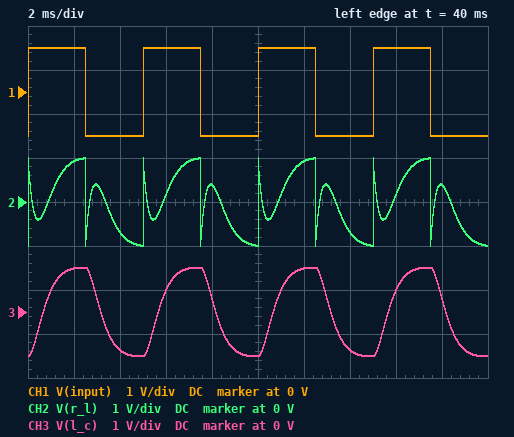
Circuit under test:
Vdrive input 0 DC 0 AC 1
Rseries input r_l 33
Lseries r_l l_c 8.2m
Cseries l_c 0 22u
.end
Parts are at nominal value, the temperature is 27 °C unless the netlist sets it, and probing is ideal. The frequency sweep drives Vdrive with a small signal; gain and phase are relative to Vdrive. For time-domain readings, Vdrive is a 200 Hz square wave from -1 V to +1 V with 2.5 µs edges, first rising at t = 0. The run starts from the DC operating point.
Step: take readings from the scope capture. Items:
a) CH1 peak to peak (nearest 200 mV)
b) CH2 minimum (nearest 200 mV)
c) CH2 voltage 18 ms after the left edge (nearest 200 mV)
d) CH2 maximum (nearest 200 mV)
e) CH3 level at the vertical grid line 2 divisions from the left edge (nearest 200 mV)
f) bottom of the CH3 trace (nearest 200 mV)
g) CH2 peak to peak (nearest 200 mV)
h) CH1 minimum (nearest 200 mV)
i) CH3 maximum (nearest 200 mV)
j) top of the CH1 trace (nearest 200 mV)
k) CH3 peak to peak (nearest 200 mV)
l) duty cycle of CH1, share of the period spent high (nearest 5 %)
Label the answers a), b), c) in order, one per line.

a) 2.0 V
b) -1.0 V
c) 400 mV
d) 1.0 V
e) -800 mV
f) -1.0 V
g) 2.0 V
h) -1.0 V
i) 1.0 V
j) 1.0 V
k) 2.0 V
l) 50 %
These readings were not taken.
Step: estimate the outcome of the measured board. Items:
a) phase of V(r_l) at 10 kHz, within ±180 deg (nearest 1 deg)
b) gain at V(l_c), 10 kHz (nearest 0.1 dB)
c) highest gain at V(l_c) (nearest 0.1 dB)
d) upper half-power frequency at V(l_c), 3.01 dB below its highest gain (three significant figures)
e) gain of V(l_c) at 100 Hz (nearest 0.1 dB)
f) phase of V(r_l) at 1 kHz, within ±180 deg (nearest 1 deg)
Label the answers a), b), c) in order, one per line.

a) 4 deg
b) -57.1 dB
c) 0 dB
d) 300 Hz
e) -0.3 dB
f) 37 deg
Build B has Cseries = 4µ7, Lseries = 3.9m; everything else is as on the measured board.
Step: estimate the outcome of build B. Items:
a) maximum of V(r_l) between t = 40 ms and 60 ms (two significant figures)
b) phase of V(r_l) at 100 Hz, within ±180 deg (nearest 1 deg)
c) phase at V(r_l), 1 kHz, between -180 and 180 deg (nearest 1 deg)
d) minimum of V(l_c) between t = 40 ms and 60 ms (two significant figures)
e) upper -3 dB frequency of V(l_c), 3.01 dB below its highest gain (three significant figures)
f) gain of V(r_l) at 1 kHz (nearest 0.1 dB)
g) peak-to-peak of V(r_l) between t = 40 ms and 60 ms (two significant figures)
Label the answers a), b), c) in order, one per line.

a) 1.1 V
b) -6 deg
c) -74 deg
d) -1.2 V
e) 1.33 kHz
f) -11.3 dB
g) 2.3 V
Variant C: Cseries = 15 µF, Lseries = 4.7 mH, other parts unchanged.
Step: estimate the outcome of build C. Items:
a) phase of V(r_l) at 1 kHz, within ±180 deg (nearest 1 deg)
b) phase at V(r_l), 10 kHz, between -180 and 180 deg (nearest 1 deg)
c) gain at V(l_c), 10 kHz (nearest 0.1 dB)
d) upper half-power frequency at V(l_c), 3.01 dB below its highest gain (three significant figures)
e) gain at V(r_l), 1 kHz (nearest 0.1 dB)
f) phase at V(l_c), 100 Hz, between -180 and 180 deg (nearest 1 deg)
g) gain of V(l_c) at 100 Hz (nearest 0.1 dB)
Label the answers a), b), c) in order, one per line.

a) 60 deg
b) 6 deg
c) -48.9 dB
d) 426 Hz
e) -6.1 dB
f) -18 deg
g) -0.2 dB
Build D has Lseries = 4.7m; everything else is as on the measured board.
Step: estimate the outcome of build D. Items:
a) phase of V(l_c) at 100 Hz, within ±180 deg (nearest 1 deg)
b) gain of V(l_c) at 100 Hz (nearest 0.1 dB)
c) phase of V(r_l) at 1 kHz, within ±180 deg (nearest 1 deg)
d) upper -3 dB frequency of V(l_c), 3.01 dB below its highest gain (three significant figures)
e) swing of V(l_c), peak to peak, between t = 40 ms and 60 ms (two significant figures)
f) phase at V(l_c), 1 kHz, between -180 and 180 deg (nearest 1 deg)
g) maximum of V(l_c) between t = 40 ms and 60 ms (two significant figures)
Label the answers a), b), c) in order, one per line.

a) -25 deg
b) -0.5 dB
c) 56 deg
d) 269 Hz
e) 1.9 V
f) -124 deg
g) 970 mV
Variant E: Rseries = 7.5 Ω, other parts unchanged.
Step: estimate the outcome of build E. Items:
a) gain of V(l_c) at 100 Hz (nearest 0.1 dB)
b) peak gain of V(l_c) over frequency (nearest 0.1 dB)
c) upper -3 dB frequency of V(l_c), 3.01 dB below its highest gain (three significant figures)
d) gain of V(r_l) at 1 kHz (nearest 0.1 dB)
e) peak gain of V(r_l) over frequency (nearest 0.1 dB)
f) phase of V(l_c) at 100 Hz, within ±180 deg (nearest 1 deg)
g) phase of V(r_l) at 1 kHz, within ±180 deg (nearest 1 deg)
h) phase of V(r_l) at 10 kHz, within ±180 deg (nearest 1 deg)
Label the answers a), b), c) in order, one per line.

a) 0.6 dB
b) 8.4 dB
c) 428 Hz
d) -0.1 dB
e) 0 dB
f) -6 deg
g) 10 deg
h) 1 deg
